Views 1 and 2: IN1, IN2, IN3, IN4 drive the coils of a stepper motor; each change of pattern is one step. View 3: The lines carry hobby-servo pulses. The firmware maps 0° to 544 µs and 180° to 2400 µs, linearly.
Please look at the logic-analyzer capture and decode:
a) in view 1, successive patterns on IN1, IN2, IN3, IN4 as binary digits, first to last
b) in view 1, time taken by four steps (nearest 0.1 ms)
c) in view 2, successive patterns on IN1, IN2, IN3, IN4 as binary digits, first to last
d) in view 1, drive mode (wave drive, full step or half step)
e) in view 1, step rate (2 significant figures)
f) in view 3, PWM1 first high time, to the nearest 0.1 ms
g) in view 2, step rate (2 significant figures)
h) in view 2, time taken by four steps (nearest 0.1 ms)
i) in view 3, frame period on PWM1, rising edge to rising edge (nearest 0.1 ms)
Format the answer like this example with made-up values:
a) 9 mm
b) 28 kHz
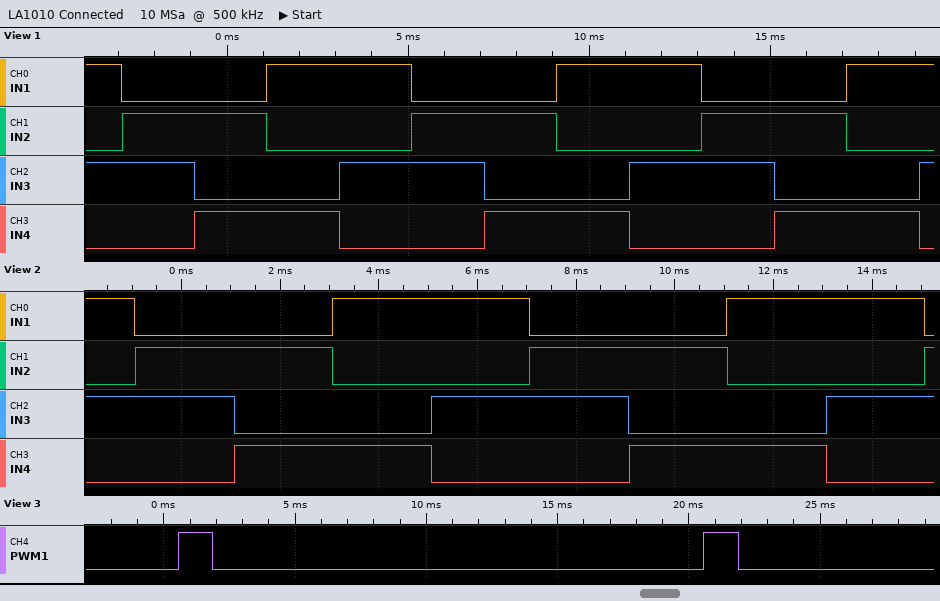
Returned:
a) 1010 0110 0101 1001 1010 0110 0101 1001 1010 0110 0101 1001 1010
b) 8.0 ms
c) 1010 0110 0101 1001 1010 0110 0101 1001 1010 0110
d) full step
e) 500 steps/s
f) 1.3 ms
g) 500 steps/s
h) 8.0 ms
i) 20.0 ms
